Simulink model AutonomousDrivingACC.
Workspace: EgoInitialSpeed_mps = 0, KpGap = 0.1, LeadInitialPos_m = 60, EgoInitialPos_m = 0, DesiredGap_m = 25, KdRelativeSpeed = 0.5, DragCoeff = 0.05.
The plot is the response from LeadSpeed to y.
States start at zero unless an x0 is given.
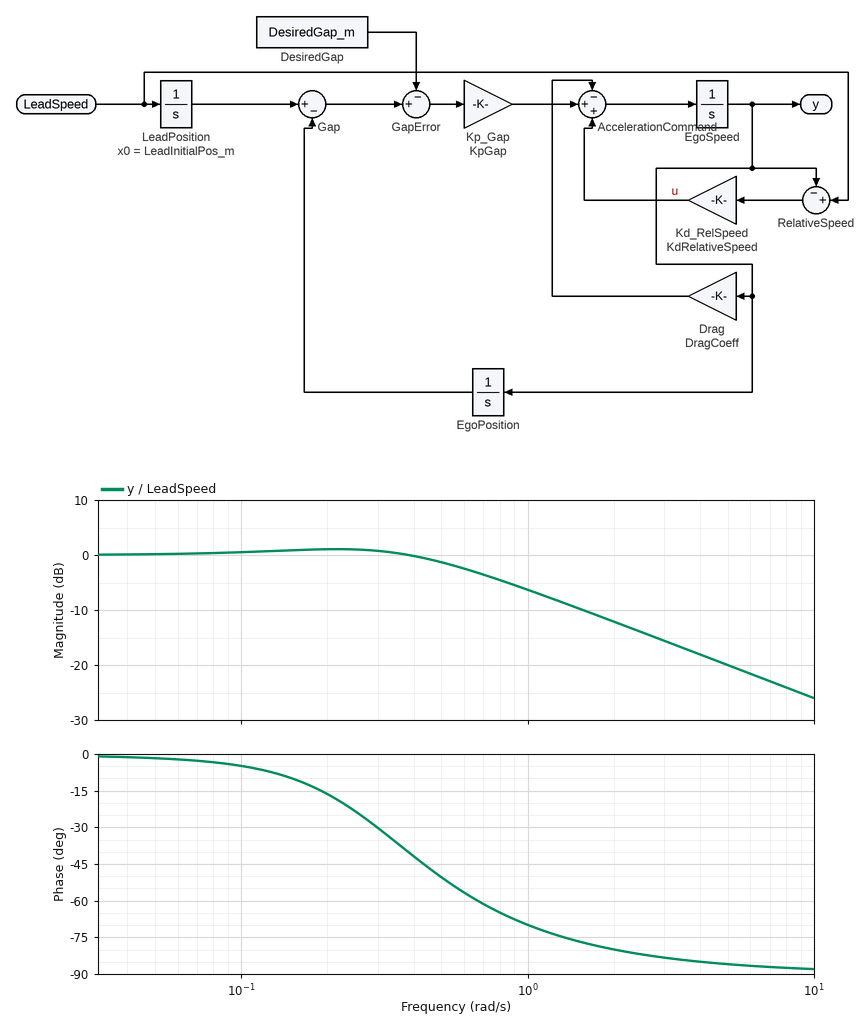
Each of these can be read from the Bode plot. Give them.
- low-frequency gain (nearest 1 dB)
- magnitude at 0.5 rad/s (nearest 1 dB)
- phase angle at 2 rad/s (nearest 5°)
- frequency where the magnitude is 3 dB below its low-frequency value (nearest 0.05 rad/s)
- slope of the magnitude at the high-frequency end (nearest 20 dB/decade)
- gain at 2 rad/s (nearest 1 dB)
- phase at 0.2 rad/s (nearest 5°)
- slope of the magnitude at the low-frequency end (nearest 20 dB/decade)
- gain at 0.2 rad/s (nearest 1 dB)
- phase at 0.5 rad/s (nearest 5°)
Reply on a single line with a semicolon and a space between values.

0 dB; -1 dB; -80°; 0.65 rad/s; -20 dB/decade; -12 dB; -15°; 0 dB/decade; 1 dB; -50°
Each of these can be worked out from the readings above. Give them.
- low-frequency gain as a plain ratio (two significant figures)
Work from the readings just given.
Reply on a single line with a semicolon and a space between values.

1.0
